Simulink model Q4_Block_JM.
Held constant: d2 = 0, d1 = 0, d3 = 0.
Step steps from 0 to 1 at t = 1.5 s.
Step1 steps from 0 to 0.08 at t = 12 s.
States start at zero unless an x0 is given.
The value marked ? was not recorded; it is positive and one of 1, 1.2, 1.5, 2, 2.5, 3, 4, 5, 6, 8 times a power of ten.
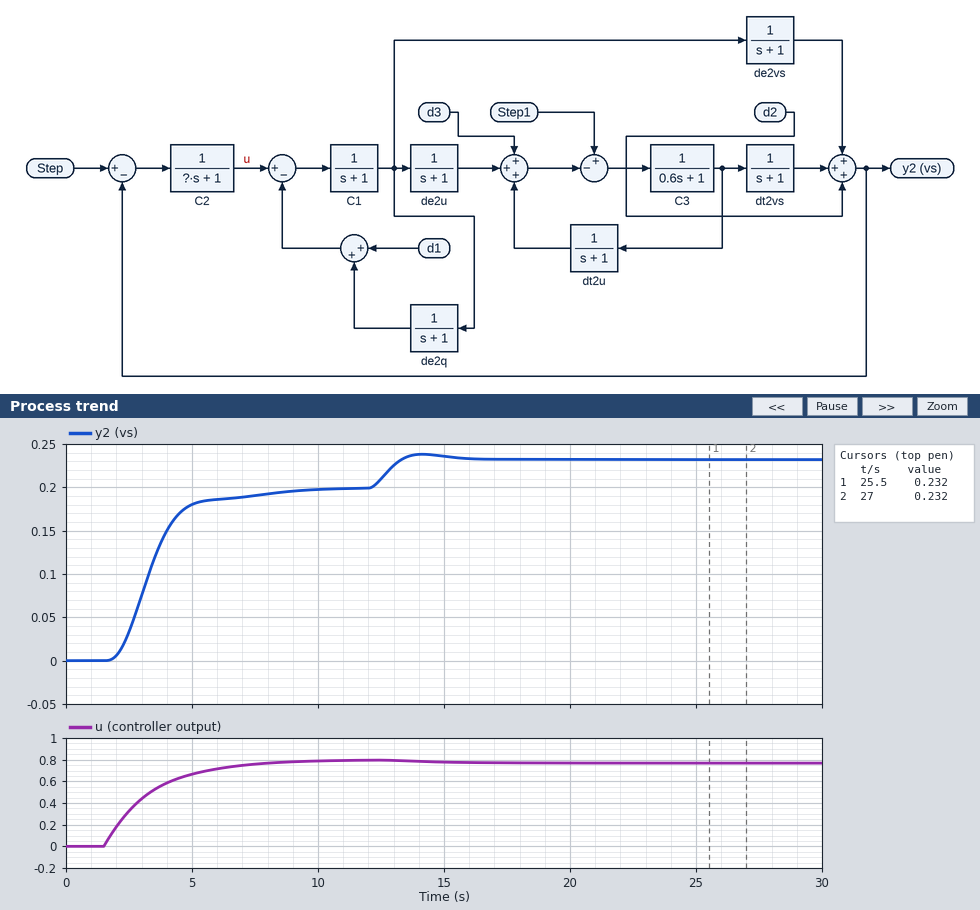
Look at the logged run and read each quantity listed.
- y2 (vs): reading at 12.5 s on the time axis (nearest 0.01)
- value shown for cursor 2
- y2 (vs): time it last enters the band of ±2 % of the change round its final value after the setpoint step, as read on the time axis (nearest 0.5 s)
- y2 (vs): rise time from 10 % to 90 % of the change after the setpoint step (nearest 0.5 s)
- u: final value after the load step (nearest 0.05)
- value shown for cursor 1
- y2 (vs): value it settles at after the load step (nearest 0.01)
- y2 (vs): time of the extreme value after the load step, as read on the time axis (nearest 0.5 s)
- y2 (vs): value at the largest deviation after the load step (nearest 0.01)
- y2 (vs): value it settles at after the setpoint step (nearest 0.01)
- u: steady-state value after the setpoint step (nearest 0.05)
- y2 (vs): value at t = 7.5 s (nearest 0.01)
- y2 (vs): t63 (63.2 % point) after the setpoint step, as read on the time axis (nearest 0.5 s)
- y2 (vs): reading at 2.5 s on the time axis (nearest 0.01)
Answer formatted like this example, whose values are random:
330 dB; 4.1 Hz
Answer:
0.21; 0.232; 9.0 s; 2.5 s; 0.75; 0.232; 0.23; 14.0 s; 0.24; 0.20; 0.80; 0.19; 3.5 s; 0.03
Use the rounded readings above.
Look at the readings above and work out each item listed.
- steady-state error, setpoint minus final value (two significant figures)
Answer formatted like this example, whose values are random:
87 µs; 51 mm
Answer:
0.80
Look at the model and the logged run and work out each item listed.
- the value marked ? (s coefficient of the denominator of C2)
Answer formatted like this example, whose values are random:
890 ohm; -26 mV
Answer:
2.5
